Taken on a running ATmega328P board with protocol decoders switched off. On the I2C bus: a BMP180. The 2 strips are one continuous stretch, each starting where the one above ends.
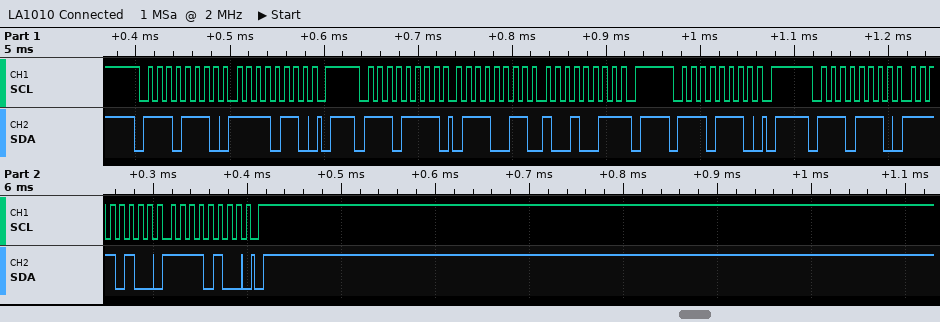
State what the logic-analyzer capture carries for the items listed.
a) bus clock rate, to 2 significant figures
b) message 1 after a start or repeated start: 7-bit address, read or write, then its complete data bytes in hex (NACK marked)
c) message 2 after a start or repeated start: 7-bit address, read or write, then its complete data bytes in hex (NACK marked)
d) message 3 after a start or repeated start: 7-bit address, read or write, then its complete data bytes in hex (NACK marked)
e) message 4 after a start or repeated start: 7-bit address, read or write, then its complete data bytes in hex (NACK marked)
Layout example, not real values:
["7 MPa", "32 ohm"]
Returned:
["100 kHz", "0x77 write: F6", "0x77 read: 73 93 NACK", "0x77 write", "0x77 write: F4 F4"]
